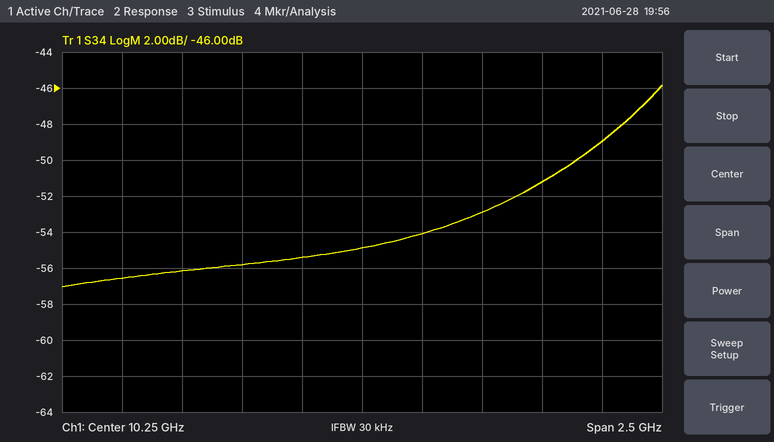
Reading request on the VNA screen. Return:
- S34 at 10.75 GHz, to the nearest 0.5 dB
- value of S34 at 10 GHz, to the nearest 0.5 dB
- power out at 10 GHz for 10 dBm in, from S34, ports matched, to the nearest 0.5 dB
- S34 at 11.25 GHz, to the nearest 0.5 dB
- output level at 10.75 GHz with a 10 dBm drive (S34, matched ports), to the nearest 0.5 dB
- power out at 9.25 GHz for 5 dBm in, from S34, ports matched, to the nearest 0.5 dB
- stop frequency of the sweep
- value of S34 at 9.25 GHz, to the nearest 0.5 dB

-53.0 dB
-55.5 dB
-45.5 dBm
-49.0 dB
-43.0 dBm
-51.5 dBm
11.5 GHz
-56.5 dB
